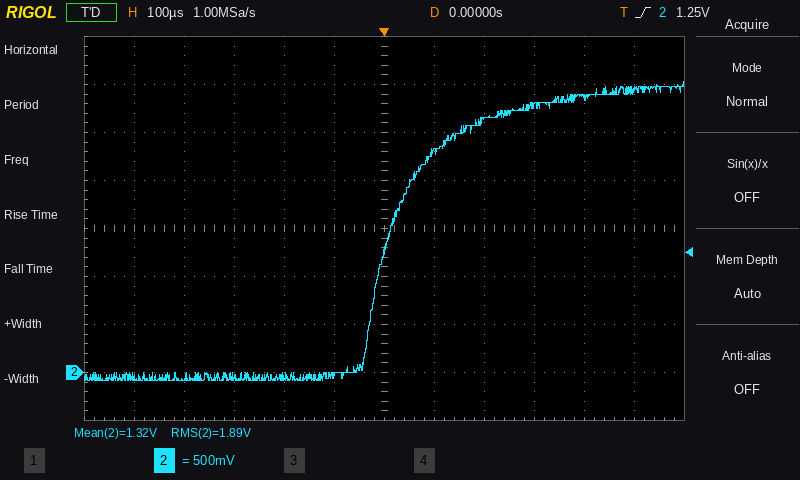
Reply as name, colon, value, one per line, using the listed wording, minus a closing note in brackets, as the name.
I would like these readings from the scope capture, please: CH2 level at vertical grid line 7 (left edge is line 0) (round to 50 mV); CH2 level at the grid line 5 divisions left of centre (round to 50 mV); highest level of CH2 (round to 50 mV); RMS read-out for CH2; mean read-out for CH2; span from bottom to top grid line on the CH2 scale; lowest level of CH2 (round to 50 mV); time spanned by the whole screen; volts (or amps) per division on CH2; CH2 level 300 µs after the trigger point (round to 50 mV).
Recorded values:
CH2 level at vertical grid line 7 (left edge is line 0): 2.30 V
CH2 level at the grid line 5 divisions left of centre: -50 mV
highest level of CH2: 3.05 V
RMS read-out for CH2: 1.89 V
mean read-out for CH2: 1.32 V
span from bottom to top grid line on the CH2 scale: 4 V
lowest level of CH2: -100 mV
time spanned by the whole screen: 1.2 ms
volts (or amps) per division on CH2: 500 mV
CH2 level 300 µs after the trigger point: 2.80 V
